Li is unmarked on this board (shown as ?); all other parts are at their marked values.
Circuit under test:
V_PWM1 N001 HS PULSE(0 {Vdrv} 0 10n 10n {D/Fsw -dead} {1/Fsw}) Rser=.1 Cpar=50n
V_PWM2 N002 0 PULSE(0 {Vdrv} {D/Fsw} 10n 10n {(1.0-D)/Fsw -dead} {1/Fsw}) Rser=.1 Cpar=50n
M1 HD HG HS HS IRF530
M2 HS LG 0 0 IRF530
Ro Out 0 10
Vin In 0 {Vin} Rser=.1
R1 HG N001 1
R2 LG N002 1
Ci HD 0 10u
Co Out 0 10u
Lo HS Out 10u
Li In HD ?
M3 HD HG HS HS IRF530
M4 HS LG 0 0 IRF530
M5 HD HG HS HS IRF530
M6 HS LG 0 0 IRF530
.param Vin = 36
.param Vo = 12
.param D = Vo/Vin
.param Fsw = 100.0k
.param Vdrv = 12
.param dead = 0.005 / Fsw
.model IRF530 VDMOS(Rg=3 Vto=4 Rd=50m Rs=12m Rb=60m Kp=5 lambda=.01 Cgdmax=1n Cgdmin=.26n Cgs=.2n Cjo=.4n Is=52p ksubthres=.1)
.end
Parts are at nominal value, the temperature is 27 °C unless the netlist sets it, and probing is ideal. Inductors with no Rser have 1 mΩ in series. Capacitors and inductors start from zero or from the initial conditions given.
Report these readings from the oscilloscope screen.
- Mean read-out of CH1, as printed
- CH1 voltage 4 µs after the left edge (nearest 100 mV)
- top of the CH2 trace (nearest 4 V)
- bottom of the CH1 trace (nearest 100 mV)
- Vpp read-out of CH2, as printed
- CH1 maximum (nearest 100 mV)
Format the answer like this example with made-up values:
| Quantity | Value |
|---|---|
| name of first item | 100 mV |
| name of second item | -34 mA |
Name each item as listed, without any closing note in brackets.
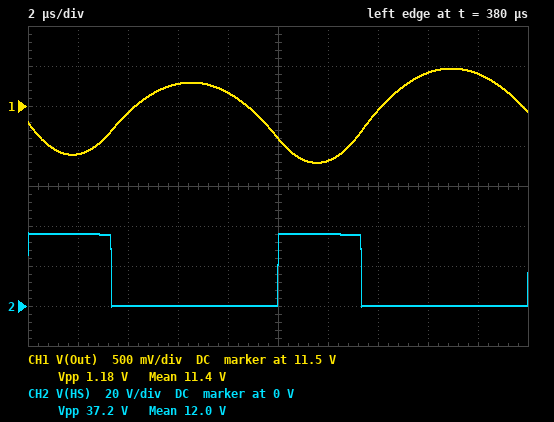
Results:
| Quantity | Value |
|---|---|
| Mean read-out of CH1, as printed | 11.4 V |
| CH1 voltage 4 µs after the left edge | 11.4 V |
| top of the CH2 trace | 36 V |
| bottom of the CH1 trace | 10.8 V |
| Vpp read-out of CH2, as printed | 37.2 V |
| CH1 maximum | 12.0 V |
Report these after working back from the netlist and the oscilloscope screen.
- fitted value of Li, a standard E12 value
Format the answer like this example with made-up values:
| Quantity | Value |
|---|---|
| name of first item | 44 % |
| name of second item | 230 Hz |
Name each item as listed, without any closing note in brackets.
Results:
| Quantity | Value |
|---|---|
| fitted value of Li, a standard E12 value | 3.3 µH |
